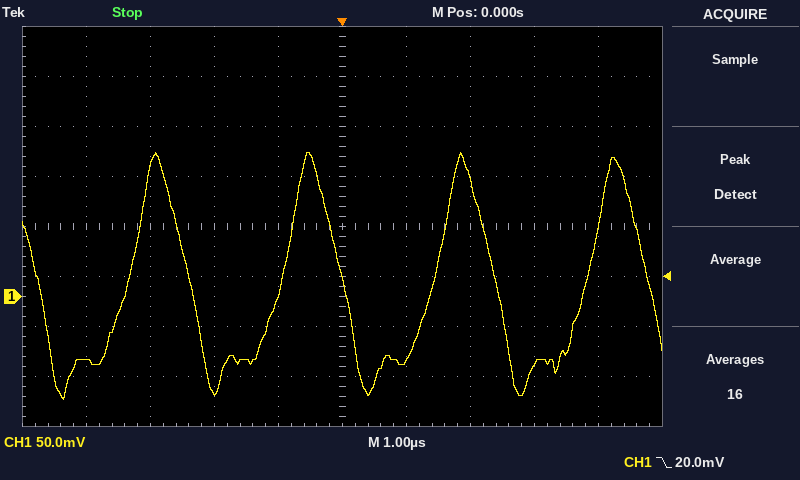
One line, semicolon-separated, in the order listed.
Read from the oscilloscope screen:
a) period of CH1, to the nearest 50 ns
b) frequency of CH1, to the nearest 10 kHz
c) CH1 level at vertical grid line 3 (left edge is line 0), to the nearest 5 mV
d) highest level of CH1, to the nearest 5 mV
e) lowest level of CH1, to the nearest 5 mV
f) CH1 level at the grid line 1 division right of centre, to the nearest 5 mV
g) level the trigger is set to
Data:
2.40 µs; 420 kHz; -95 mV; 145 mV; -105 mV; -65 mV; 20.0 mV
